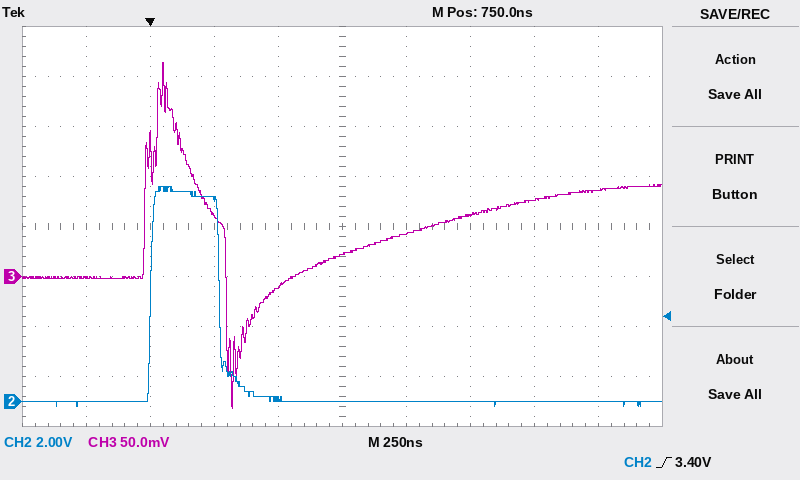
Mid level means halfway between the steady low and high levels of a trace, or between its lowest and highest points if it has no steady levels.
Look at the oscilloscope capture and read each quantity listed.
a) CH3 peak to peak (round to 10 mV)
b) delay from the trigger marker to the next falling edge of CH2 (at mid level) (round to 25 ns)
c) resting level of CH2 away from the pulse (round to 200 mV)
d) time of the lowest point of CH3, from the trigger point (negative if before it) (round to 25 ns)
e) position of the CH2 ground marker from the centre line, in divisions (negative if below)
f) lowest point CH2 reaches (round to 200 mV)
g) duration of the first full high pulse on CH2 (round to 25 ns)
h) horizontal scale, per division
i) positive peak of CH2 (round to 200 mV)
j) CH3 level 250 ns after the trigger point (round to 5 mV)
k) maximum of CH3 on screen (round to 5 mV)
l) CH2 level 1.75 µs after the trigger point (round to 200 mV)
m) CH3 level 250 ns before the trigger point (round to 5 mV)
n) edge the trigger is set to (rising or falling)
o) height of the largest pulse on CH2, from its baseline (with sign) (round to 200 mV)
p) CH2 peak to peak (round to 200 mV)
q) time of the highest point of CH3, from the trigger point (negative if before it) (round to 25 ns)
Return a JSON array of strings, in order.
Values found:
["350 mV", "275 ns", "0.0 V", "+325 ns", "-3.5 div", "-200 mV", "275 ns", "250 ns", "8.6 V", "60 mV", "215 mV", "0.0 V", "0 mV", "rising", "+8.6 V", "8.8 V", "+50 ns"]
